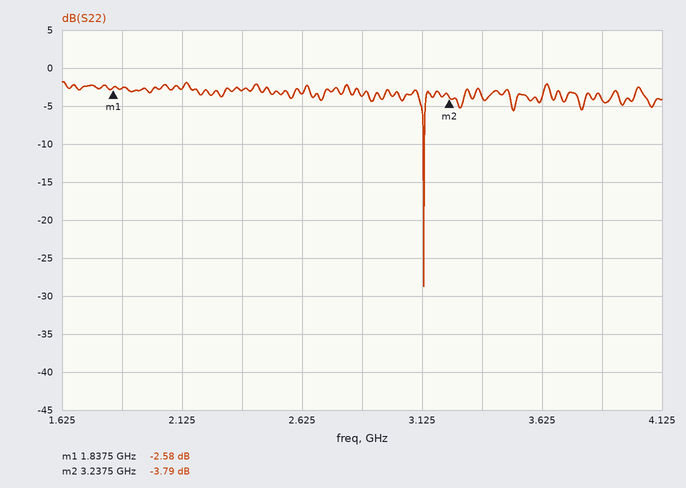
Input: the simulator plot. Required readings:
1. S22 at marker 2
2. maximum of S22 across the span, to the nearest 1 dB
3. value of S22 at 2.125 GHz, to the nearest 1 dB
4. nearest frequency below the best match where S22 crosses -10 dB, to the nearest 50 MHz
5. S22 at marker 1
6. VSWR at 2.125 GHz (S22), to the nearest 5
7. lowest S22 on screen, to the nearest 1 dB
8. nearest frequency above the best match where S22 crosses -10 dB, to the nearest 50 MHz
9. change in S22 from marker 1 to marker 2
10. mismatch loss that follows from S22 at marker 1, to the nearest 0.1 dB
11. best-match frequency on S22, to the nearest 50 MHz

-3.79 dB
-2 dB
-3 dB
3.15 GHz
-2.58 dB
5
-29 dB
3.15 GHz
-1.21 dB
3.5 dB
3.15 GHz
